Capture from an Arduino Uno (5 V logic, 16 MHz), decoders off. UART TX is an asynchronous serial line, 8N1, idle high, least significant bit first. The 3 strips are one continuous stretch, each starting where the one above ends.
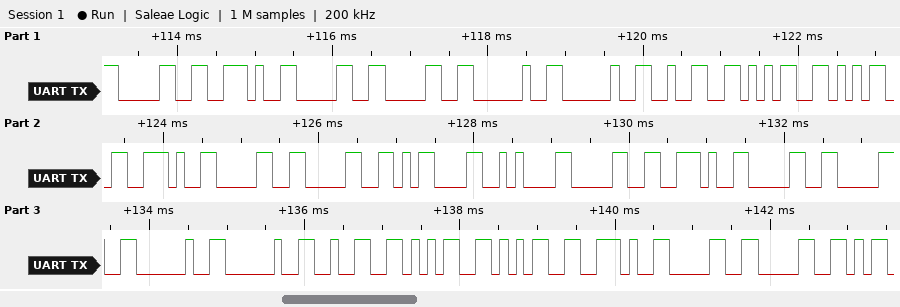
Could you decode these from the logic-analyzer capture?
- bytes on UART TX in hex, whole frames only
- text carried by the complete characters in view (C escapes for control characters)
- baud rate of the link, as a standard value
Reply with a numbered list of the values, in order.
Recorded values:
1. 30 2E 30 30 20 20 32 35 35 2E 30 30 0D 0A 30 2E 30 30 20 20 32 35 35 2E 30 30
2. "0.00  255.00\r\n0.00  255.00"
3. 9600 baud
